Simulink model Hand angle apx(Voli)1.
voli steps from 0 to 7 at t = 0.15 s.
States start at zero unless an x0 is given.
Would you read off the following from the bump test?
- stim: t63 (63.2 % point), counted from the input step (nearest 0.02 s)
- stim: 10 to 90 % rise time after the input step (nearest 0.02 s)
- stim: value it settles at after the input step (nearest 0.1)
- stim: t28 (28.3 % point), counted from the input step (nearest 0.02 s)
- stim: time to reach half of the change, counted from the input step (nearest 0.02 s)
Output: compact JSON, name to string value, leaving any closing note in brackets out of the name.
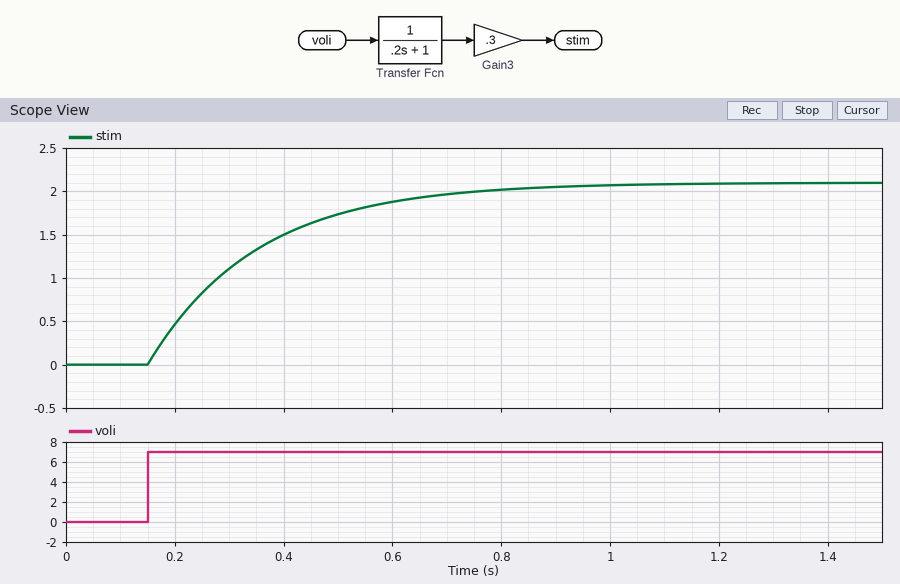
{"stim: t63 (63.2 % point), counted from the input step": "0.20 s", "stim: 10 to 90 % rise time after the input step": "0.44 s", "stim: value it settles at after the input step": "2.1", "stim: t28 (28.3 % point), counted from the input step": "0.06 s", "stim: time to reach half of the change, counted from the input step": "0.14 s"}
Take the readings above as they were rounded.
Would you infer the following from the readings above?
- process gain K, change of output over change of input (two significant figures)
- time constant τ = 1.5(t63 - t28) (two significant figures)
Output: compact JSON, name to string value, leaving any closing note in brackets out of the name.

{"process gain K, change of output over change of input": "0.30", "time constant τ = 1.5(t63 - t28)": "0.21 s"}
